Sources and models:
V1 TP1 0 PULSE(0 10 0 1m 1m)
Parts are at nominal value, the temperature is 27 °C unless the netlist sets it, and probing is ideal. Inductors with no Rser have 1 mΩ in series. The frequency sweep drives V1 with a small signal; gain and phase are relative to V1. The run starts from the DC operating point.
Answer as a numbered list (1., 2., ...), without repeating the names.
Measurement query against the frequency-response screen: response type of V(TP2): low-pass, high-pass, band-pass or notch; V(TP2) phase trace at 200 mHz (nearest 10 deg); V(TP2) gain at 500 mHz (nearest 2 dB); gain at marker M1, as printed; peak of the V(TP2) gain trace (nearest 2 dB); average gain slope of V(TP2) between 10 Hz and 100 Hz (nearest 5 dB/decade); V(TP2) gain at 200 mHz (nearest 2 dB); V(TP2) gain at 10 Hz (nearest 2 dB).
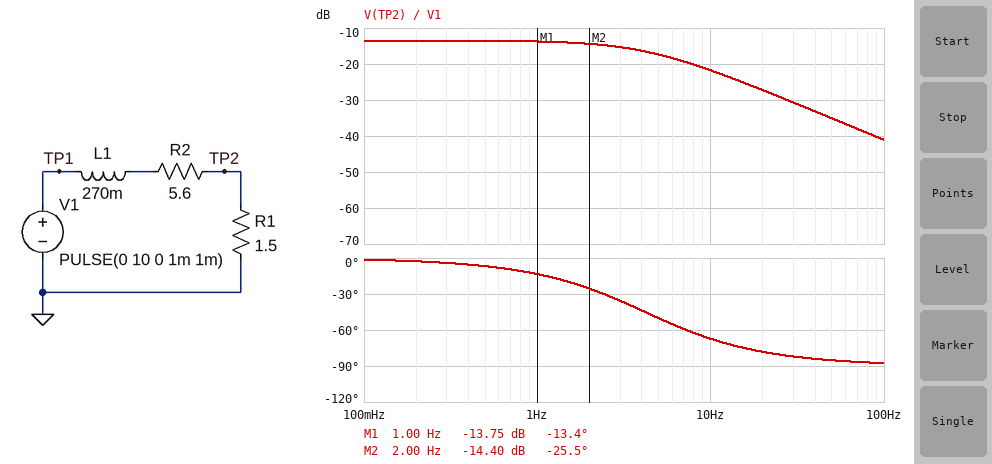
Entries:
1. low-pass
2. 0 deg
3. -14 dB
4. -13.75 dB
5. -14 dB
6. -20 dB/decade
7. -14 dB
8. -22 dB
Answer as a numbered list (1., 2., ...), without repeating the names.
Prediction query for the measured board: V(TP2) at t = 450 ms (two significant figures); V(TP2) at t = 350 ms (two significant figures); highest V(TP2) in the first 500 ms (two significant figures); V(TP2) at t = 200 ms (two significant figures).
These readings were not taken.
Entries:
1. 2.1 V
2. 2.1 V
3. 2.1 V
4. 2.1 V
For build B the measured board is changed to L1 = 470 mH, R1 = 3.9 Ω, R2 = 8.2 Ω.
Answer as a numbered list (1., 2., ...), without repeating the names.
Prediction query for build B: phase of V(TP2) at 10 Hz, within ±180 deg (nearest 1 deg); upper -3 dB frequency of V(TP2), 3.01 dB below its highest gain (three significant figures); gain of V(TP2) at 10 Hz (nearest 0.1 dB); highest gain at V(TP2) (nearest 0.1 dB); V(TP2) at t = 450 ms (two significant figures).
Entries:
1. -68 deg
2. 4.10 Hz
3. -18.3 dB
4. -9.8 dB
5. 3.2 V
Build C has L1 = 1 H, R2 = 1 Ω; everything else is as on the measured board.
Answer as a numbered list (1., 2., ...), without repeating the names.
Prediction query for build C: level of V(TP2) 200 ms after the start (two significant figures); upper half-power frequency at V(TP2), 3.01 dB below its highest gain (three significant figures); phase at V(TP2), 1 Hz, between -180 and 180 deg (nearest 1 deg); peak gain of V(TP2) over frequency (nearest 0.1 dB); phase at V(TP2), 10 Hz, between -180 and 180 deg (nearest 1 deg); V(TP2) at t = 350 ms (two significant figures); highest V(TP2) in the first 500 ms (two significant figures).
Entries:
1. 2.4 V
2. 398 mHz
3. -68 deg
4. -4.4 dB
5. -88 deg
6. 3.5 V
7. 4.3 V
